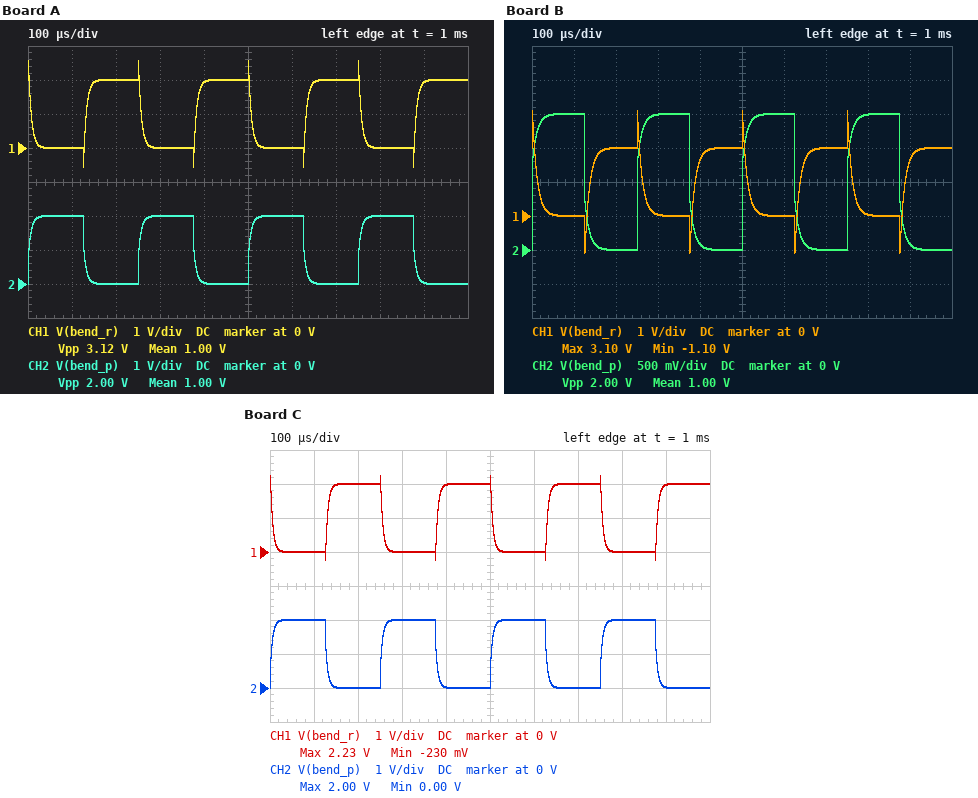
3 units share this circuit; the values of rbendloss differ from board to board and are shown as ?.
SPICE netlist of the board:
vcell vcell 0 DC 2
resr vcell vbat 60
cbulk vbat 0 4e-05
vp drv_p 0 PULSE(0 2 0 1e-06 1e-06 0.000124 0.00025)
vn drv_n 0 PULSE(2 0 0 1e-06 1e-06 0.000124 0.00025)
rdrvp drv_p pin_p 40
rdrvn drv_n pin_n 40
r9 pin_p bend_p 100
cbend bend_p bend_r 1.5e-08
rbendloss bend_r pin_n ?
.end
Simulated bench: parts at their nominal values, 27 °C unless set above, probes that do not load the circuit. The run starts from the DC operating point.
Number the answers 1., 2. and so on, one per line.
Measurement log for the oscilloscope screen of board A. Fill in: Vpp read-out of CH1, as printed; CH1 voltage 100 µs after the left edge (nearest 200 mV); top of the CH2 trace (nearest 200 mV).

1. 3.12 V
2. 0 V
3. 2.0 V
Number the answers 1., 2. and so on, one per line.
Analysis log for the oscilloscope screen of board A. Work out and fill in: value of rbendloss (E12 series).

1. 270 Ω
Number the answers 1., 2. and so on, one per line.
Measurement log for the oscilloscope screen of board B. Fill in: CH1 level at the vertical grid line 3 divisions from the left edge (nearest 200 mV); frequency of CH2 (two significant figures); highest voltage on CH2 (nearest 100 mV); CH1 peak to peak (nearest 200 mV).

1. 0 V
2. 4.0 kHz
3. 2.0 V
4. 4.2 V
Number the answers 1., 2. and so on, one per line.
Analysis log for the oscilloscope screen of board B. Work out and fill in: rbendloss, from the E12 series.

1. 560 Ω
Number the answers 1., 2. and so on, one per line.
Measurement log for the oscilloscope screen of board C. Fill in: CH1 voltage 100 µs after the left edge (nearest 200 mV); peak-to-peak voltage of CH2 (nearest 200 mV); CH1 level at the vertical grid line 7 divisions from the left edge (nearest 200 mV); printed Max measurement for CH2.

1. 0 V
2. 2.0 V
3. 2.0 V
4. 2.00 V
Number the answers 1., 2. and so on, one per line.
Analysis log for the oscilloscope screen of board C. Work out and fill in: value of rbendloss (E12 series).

1. 180 Ω
